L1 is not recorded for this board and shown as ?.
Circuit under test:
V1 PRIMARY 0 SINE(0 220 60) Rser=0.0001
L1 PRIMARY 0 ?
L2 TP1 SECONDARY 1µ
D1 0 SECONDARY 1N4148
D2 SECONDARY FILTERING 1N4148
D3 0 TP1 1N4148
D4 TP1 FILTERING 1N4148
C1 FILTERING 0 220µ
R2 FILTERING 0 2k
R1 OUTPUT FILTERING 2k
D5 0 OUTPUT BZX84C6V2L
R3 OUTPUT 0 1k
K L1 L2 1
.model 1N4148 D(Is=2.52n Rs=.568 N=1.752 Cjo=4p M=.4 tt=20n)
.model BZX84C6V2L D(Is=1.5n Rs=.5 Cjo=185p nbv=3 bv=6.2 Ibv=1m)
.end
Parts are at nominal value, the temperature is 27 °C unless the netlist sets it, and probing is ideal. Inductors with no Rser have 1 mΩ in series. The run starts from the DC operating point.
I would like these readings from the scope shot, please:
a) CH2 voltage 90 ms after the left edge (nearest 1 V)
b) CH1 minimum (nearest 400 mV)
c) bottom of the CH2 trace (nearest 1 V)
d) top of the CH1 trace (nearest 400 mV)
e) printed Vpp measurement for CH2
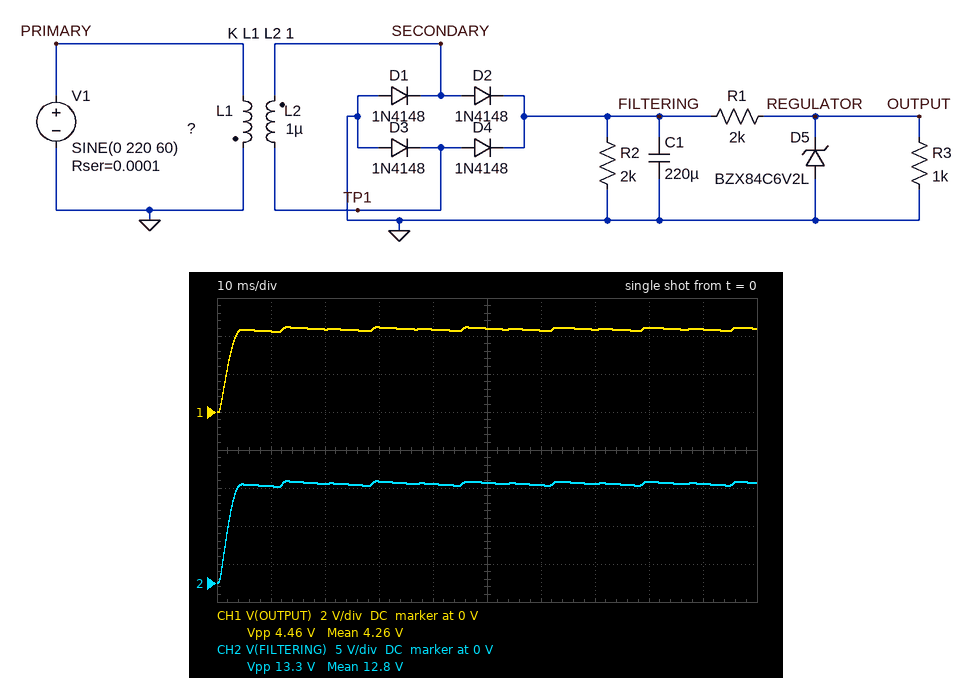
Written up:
13 V
0 V
0 V
4.4 V
13.3 V
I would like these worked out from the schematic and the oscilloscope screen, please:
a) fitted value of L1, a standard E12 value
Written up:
220 µH
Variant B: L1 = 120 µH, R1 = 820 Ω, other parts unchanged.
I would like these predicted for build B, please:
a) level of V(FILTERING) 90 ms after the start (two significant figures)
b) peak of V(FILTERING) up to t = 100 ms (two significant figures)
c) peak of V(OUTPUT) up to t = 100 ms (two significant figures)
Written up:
18 V
19 V
6.4 V
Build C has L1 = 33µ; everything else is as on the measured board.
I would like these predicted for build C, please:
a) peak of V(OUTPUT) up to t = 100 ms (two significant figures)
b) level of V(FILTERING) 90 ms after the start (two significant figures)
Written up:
6.4 V
36 V
